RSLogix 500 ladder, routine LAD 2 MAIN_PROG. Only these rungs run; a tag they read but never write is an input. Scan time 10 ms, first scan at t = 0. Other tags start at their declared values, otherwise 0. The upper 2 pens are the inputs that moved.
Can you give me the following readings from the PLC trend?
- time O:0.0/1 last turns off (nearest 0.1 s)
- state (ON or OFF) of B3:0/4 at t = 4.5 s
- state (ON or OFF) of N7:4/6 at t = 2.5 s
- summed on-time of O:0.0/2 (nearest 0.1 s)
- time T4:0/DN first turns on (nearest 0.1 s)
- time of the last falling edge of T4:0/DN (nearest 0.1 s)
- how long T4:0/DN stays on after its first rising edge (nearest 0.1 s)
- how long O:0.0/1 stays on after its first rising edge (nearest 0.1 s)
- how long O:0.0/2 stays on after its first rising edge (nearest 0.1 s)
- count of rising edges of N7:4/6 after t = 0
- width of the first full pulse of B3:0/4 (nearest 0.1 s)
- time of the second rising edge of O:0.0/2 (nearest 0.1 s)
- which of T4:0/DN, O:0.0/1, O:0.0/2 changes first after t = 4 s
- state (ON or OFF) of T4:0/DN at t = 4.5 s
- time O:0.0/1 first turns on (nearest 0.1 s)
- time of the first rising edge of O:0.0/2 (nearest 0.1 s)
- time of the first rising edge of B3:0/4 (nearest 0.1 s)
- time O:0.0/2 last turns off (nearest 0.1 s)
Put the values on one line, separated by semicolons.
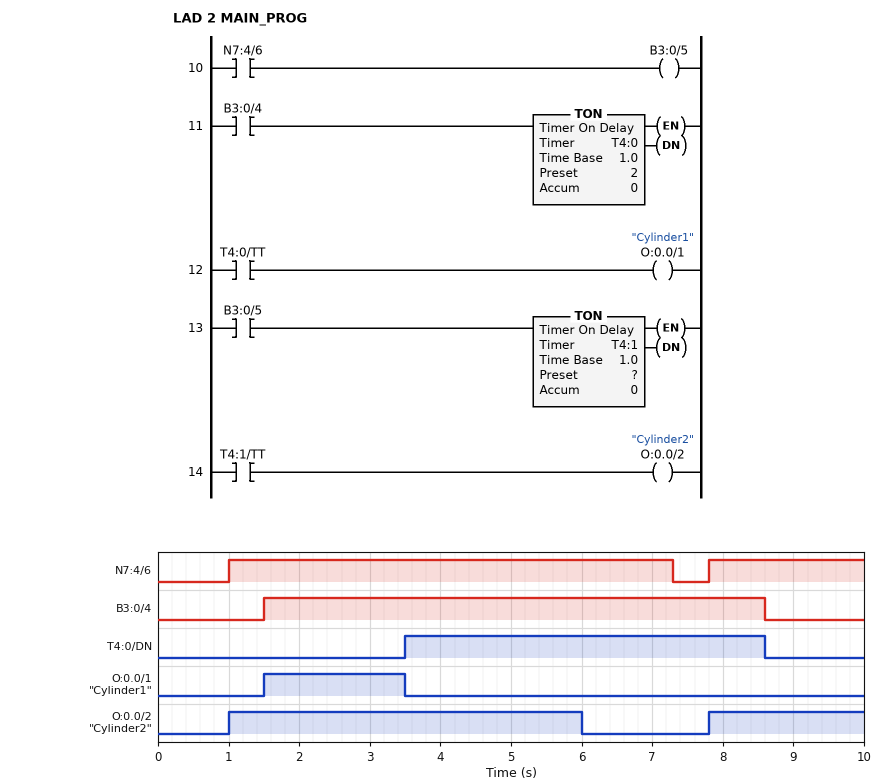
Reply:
3.5 s; ON; ON; 7.2 s; 3.5 s; 8.6 s; 5.1 s; 2.0 s; 5.0 s; 2; 7.1 s; 7.8 s; O:0.0/2; ON; 1.5 s; 1.0 s; 1.5 s; 6.0 s
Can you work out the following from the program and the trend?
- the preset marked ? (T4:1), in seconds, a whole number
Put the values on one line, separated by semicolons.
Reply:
5 s
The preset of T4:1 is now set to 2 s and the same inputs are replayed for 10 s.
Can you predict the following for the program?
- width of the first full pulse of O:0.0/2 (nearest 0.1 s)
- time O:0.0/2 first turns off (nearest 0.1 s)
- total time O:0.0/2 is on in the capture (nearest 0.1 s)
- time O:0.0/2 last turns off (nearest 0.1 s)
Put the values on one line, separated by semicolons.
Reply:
2.0 s; 3.0 s; 4.0 s; 9.8 s
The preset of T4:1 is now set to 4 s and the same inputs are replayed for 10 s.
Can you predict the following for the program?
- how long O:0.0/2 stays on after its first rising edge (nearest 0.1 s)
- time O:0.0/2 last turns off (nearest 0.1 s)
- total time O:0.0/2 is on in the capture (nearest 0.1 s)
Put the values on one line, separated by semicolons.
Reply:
4.0 s; 5.0 s; 6.2 s
